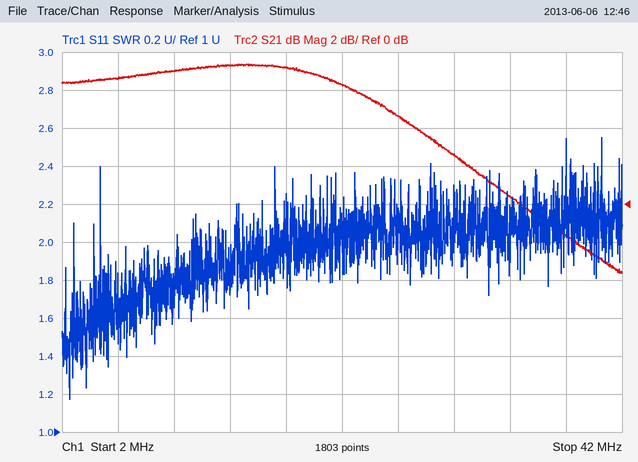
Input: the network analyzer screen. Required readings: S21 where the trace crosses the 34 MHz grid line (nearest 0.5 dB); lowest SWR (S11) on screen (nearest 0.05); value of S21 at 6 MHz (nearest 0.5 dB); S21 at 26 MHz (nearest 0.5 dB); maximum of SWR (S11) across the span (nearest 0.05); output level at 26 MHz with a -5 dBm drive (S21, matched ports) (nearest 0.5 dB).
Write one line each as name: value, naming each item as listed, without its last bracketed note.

S21 where the trace crosses the 34 MHz grid line: 0.5 dB
lowest SWR (S11) on screen: 1.15
value of S21 at 6 MHz: 6.5 dB
S21 at 26 MHz: 4.5 dB
maximum of SWR (S11) across the span: 2.55
output level at 26 MHz with a -5 dBm drive (S21, matched ports): -0.5 dBm
